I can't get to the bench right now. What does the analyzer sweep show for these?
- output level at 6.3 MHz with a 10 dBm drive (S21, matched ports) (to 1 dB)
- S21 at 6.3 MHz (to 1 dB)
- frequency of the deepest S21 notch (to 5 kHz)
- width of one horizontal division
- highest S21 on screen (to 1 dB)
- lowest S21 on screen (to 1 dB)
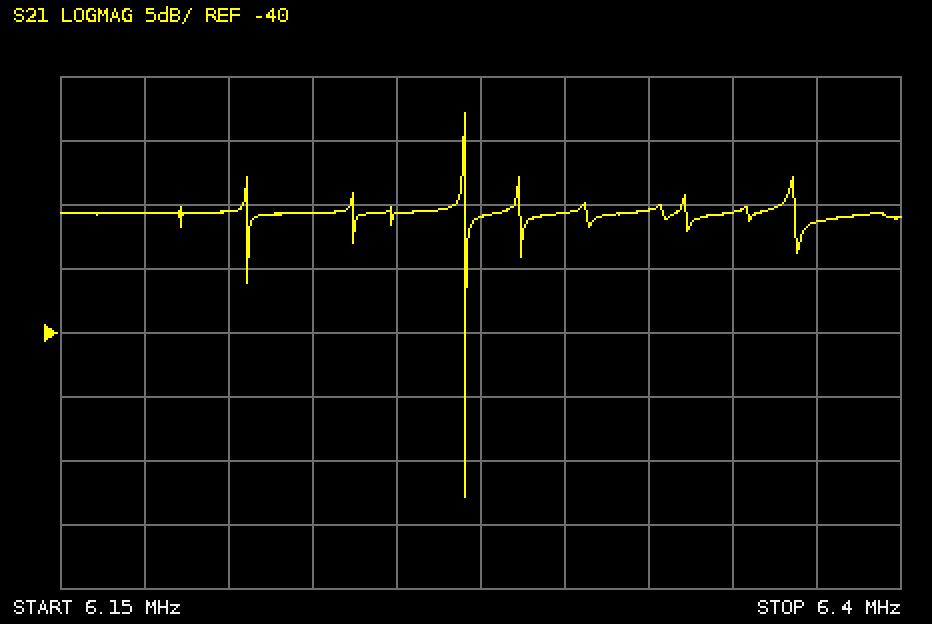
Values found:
-21 dBm
-31 dB
6.270 MHz
25 kHz
-23 dB
-53 dB
